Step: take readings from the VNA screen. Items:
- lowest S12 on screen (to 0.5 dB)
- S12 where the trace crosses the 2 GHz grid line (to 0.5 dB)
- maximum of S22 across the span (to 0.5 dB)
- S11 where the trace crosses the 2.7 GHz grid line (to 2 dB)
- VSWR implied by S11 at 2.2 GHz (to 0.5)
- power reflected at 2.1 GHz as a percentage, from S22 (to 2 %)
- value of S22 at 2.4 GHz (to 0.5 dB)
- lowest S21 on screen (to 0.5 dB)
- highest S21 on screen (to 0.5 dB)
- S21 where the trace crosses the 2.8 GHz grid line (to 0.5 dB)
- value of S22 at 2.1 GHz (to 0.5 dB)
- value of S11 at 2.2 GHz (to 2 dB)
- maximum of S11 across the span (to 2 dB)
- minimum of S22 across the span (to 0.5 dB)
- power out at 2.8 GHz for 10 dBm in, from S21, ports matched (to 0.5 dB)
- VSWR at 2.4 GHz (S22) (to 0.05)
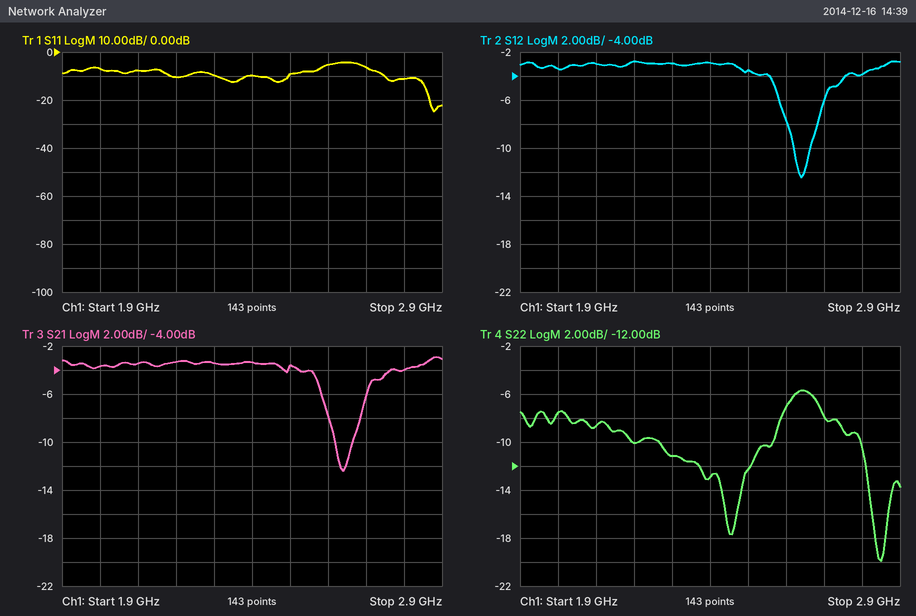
-12.5 dB
-3.5 dB
-5.5 dB
-6 dB
2.0
14 %
-13.0 dB
-12.5 dB
-3.0 dB
-4.0 dB
-8.5 dB
-10 dB
-4 dB
-20.0 dB
6.0 dBm
1.60
